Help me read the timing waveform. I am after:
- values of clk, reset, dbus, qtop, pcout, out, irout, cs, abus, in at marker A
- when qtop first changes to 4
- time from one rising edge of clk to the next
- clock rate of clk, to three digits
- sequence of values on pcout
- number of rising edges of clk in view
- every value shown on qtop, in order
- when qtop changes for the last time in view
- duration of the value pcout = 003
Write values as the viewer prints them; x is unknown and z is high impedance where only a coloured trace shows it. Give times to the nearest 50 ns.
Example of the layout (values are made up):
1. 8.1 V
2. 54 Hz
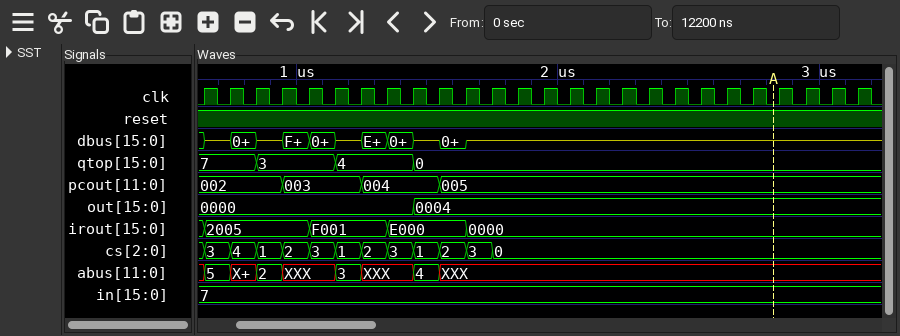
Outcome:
1. clk=0, reset=1, dbus=z, qtop=0, pcout=005, out=0004, irout=0000, cs=0, abus=XXX, in=7
2. 1150 ns
3. 100 ns
4. 10.0 MHz
5. 002, 003, 004, 005
6. 26
7. 7, 3, 4, 0
8. 1450 ns
9. 300 ns
